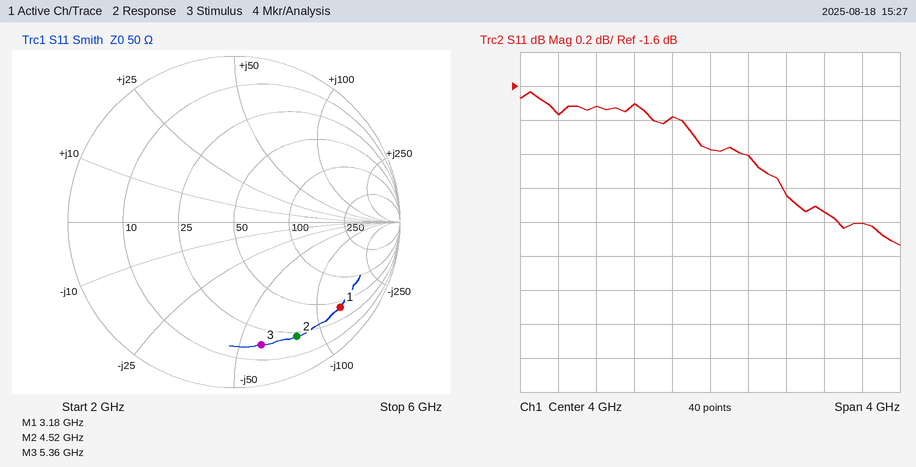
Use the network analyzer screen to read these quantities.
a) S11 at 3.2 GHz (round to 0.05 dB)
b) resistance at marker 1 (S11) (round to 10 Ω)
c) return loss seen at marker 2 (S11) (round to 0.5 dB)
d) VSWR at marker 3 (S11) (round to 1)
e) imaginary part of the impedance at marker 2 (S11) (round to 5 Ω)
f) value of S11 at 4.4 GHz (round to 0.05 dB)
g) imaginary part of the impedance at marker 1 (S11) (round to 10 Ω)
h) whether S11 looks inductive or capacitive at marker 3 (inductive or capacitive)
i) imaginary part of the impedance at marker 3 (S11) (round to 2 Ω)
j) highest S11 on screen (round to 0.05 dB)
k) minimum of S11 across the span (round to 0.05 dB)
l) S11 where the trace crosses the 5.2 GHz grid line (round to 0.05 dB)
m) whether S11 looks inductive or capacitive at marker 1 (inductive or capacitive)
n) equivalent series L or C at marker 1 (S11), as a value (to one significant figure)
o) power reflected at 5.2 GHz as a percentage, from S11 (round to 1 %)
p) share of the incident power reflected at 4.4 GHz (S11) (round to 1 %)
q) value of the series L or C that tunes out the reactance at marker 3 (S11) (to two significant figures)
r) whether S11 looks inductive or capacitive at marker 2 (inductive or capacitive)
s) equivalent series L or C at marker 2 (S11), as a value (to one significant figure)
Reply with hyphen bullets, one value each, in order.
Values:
- -1.70 dB
- 40 Ω
- 2.0 dB
- 7
- -80 Ω
- -2.00 dB
- -130 Ω
- capacitive
- -60 Ω
- -1.65 dB
- -2.55 dB
- -2.35 dB
- capacitive
- 400 fF
- 58 %
- 63 %
- 1.8 nH
- capacitive
- 400 fF
